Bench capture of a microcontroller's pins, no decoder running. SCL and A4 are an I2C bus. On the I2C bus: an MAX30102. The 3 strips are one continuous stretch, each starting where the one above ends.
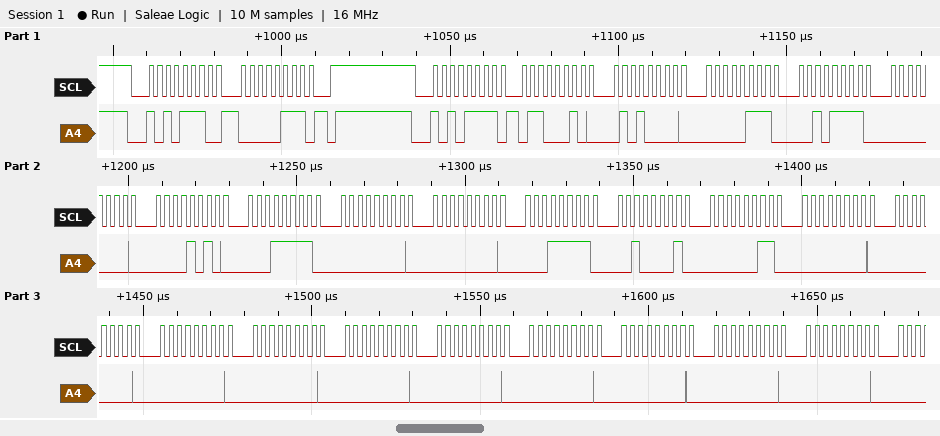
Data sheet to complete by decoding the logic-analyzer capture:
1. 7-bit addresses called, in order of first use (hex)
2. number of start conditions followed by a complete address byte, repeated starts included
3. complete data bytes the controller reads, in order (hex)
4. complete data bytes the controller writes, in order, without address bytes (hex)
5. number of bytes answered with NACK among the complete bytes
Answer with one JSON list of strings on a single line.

["0x57", "2", "62 50 07 2F 00 0A 1F 00 00 1F 21 03 00 00 00 00 00 00 00 00 00 00", "07", "0"]
